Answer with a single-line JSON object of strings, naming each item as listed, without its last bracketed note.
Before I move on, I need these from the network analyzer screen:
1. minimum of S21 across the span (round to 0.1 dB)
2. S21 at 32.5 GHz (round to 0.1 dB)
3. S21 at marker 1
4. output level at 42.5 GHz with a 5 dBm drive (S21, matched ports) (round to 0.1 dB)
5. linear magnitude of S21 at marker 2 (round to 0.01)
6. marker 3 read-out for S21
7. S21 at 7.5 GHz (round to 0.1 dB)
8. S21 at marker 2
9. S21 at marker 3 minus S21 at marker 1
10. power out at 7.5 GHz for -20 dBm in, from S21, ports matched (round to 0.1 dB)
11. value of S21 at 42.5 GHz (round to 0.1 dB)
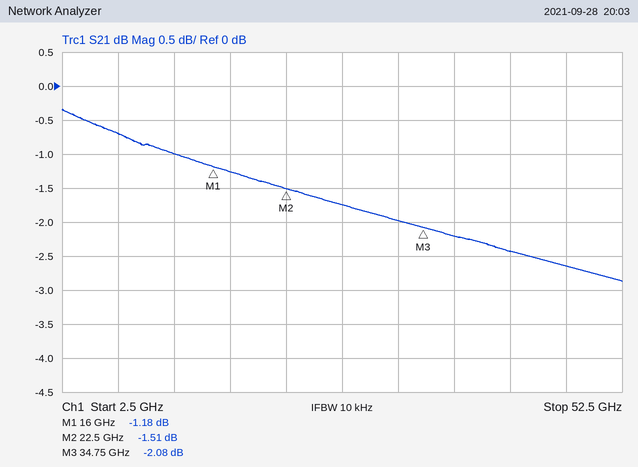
{"minimum of S21 across the span": "-2.9 dB", "S21 at 32.5 GHz": "-2.0 dB", "S21 at marker 1": "-1.18 dB", "output level at 42.5 GHz with a 5 dBm drive (S21, matched ports)": "2.6 dBm", "linear magnitude of S21 at marker 2": "0.84", "marker 3 read-out for S21": "-2.08 dB", "S21 at 7.5 GHz": "-0.7 dB", "S21 at marker 2": "-1.51 dB", "S21 at marker 3 minus S21 at marker 1": "-0.90 dB", "power out at 7.5 GHz for -20 dBm in, from S21, ports matched": "-20.7 dBm", "value of S21 at 42.5 GHz": "-2.4 dB"}
